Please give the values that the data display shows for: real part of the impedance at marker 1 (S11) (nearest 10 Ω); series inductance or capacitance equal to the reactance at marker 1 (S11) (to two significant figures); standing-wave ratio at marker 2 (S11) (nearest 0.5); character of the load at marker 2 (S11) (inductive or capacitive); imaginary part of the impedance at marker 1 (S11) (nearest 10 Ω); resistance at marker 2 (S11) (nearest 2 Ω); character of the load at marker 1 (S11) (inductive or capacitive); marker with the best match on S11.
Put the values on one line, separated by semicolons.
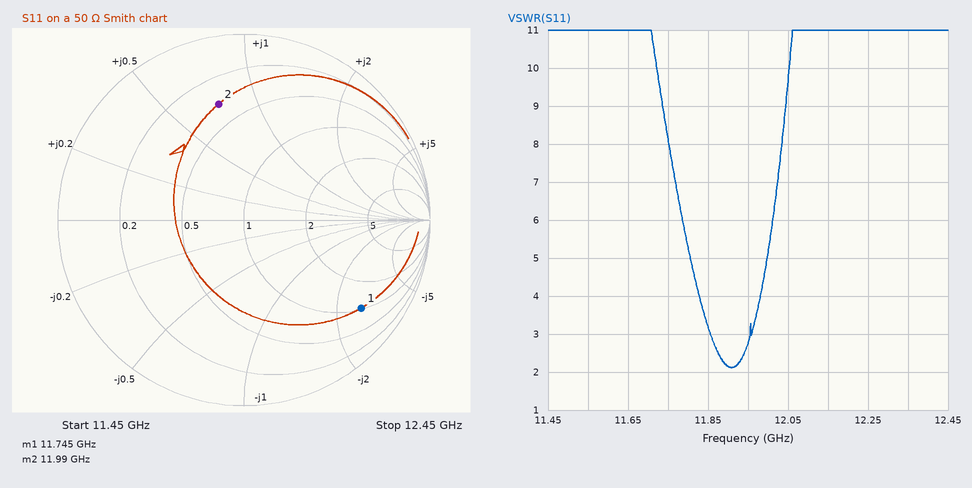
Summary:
50 Ω; 100 fF; 4.5; inductive; -130 Ω; 18 Ω; capacitive; marker 2
